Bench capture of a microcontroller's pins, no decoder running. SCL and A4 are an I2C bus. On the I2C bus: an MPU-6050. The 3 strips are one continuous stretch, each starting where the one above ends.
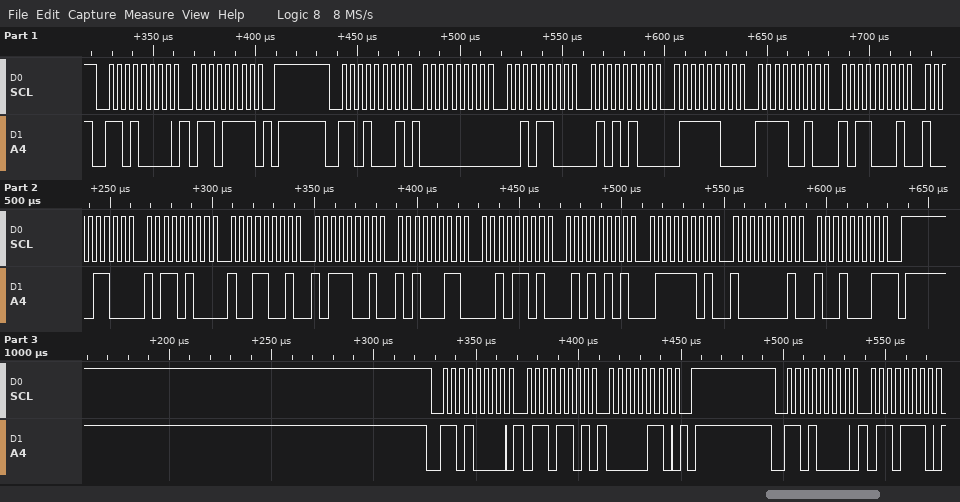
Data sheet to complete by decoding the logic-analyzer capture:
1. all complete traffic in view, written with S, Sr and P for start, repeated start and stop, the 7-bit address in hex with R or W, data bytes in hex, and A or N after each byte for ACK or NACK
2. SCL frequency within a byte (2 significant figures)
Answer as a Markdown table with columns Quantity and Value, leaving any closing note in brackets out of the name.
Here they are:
| Quantity | Value |
|---|---|
| all complete traffic in view, written with S, Sr and P for start, repeated start and stop, the 7-bit address in hex with R or W, data bytes in hex, and A or N after each byte for ACK or NACK | S 68W A 6F A P S 68R A 00 A 2C A 54 A 7C A F2 A B1 A 8C A B4 A 99 A B9 A A3 A 2D A 55 A 7D A 81 A 91 N P S 68W A 6D A 06 A P S 68W A 6E A |
| SCL frequency within a byte | 250 kHz |
